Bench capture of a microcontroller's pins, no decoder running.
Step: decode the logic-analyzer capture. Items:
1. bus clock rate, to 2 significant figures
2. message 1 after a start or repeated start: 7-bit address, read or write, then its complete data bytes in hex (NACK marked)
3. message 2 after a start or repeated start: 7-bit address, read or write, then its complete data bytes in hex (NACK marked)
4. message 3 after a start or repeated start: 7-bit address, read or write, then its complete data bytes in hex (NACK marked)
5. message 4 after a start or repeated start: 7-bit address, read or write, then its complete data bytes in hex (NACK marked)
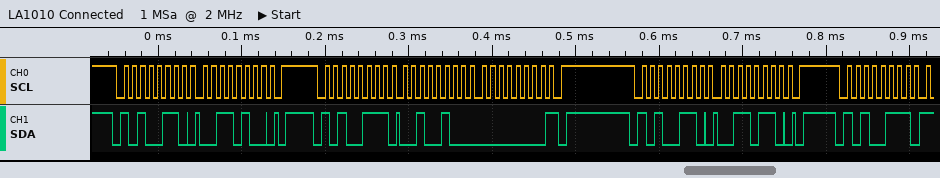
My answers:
100 kHz
0x53 write: 34
0x53 read: 24 00 NACK
0x53 write: 36
0x53 read
